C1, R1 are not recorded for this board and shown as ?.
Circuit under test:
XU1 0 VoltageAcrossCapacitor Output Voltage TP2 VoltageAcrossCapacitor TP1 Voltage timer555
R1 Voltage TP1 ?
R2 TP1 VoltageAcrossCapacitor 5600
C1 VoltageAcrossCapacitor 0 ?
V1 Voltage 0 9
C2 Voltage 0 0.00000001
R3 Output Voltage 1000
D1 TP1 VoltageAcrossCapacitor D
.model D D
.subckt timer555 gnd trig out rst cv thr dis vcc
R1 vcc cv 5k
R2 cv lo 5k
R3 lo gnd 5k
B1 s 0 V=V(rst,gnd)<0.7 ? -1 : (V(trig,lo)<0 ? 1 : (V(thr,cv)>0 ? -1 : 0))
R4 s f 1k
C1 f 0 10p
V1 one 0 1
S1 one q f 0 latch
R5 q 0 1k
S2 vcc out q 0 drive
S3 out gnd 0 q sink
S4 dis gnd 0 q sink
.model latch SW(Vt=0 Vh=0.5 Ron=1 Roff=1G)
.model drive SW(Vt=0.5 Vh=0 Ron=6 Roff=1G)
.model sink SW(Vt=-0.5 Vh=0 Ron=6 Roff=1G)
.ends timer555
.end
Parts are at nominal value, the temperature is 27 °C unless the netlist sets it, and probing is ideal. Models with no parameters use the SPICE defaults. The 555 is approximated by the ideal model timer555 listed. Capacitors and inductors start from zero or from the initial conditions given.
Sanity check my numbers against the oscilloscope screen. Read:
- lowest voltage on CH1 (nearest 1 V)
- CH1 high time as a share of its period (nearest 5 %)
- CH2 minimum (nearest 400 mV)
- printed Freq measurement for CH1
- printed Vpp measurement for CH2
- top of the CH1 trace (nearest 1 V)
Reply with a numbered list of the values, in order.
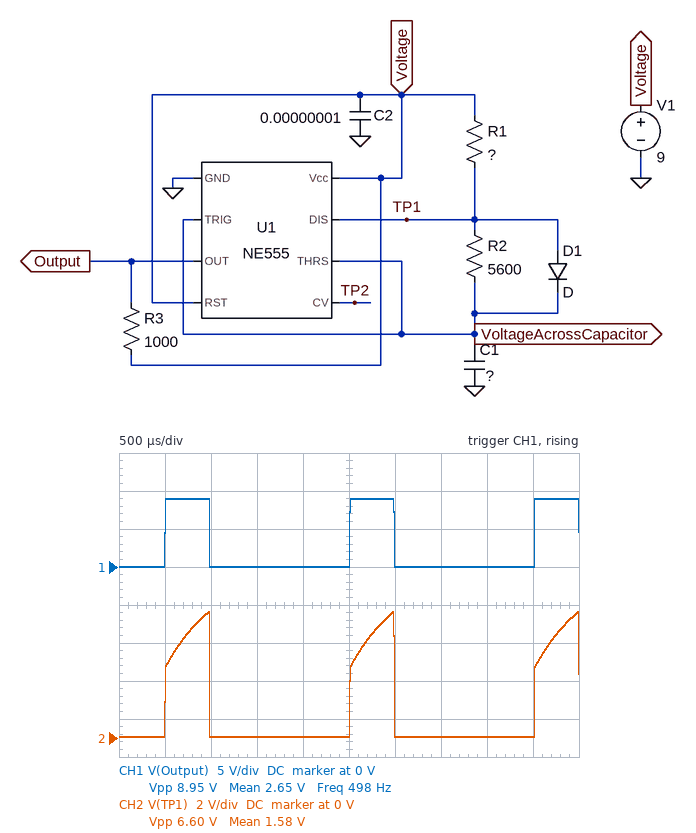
1. 0 V
2. 25 %
3. 0 V
4. 498 Hz
5. 6.60 V
6. 9 V
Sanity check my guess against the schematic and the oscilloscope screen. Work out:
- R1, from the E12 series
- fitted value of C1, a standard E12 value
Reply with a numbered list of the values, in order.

1. 1.5 kΩ
2. 390 nF
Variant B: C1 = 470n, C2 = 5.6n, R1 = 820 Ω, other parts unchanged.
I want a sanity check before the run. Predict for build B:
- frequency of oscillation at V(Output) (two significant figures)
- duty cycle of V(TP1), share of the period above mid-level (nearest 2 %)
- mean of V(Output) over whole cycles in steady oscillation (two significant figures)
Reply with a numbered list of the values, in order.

1. 460 Hz
2. 14 %
3. 1.4 V
